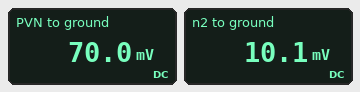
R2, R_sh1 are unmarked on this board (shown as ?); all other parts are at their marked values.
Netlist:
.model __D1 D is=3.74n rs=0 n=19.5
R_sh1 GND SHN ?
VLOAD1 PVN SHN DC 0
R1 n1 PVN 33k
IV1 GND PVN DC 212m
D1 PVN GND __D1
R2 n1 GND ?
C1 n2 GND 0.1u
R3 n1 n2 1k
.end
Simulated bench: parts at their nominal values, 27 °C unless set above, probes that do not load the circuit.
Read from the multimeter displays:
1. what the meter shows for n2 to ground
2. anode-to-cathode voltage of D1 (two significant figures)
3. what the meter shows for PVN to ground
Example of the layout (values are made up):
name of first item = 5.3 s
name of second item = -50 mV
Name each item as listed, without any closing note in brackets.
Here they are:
what the meter shows for n2 to ground = 10.1 mV
anode-to-cathode voltage of D1 = 70 mV
what the meter shows for PVN to ground = 70.0 mV
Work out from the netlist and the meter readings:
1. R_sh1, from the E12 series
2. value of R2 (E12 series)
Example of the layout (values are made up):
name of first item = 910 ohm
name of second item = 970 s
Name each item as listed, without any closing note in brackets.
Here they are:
R_sh1, from the E12 series = 0.33 Ω
value of R2 = 5.6 kΩ
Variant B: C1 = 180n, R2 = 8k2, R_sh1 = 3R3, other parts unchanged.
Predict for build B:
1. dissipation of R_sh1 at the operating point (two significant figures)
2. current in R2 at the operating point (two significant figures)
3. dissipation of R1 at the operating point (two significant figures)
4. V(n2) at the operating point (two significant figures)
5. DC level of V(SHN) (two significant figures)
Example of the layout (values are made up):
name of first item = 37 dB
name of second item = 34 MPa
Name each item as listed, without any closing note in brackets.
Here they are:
dissipation of R_sh1 at the operating point = 150 mW
current in R2 at the operating point = 17 µA
dissipation of R1 at the operating point = 9.5 µW
V(n2) at the operating point = 140 mV
DC level of V(SHN) = 700 mV
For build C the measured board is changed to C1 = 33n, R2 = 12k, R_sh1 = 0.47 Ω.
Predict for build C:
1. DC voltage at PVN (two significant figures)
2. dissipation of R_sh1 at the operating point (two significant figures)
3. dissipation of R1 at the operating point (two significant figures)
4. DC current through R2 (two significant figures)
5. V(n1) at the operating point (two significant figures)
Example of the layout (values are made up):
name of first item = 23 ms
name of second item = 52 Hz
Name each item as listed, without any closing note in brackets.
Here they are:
DC voltage at PVN = 100 mV
dissipation of R_sh1 at the operating point = 21 mW
dissipation of R1 at the operating point = 160 nW
DC current through R2 = 2.2 µA
V(n1) at the operating point = 27 mV
